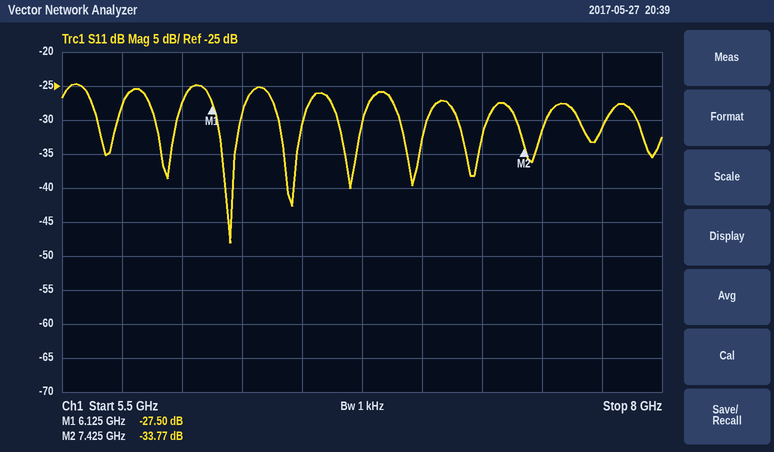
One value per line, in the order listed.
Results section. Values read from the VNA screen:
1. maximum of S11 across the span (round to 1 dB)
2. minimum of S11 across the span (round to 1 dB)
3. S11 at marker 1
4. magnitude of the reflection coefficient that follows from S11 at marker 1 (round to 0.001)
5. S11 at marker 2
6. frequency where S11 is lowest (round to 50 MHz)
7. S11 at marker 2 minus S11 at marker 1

-25 dB
-48 dB
-27.50 dB
0.042
-33.77 dB
6.20 GHz
-6.27 dB
